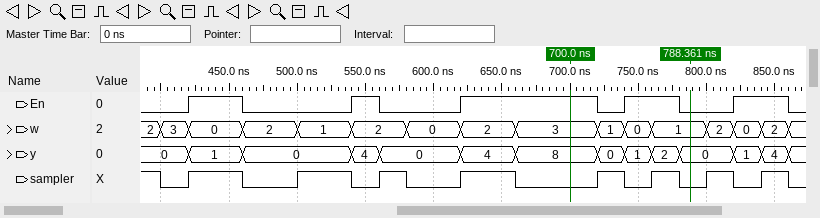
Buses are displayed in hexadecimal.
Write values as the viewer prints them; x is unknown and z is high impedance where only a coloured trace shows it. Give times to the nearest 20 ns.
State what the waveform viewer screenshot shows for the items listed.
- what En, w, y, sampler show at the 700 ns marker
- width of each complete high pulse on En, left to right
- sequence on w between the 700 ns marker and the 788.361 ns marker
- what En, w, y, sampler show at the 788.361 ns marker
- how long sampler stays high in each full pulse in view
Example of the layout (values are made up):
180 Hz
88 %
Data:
En=1, w=3, y=8, sampler=0
40 ns, 20 ns, 100 ns, 40 ns, 40 ns
3, 1, 0, 1
En=0, w=1, y=0, sampler=0
40 ns, 40 ns, 20 ns, 40 ns, 20 ns, 20 ns, 20 ns, 20 ns
